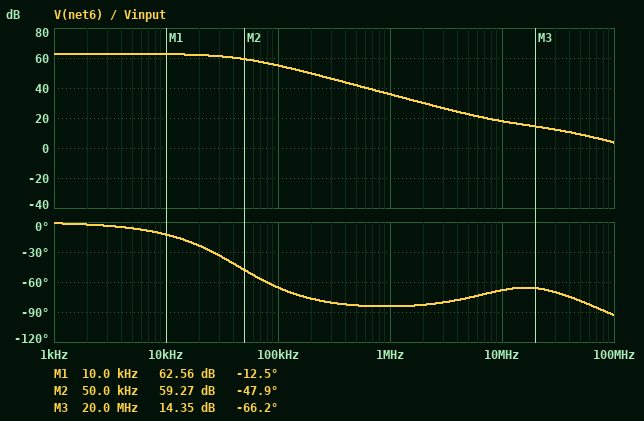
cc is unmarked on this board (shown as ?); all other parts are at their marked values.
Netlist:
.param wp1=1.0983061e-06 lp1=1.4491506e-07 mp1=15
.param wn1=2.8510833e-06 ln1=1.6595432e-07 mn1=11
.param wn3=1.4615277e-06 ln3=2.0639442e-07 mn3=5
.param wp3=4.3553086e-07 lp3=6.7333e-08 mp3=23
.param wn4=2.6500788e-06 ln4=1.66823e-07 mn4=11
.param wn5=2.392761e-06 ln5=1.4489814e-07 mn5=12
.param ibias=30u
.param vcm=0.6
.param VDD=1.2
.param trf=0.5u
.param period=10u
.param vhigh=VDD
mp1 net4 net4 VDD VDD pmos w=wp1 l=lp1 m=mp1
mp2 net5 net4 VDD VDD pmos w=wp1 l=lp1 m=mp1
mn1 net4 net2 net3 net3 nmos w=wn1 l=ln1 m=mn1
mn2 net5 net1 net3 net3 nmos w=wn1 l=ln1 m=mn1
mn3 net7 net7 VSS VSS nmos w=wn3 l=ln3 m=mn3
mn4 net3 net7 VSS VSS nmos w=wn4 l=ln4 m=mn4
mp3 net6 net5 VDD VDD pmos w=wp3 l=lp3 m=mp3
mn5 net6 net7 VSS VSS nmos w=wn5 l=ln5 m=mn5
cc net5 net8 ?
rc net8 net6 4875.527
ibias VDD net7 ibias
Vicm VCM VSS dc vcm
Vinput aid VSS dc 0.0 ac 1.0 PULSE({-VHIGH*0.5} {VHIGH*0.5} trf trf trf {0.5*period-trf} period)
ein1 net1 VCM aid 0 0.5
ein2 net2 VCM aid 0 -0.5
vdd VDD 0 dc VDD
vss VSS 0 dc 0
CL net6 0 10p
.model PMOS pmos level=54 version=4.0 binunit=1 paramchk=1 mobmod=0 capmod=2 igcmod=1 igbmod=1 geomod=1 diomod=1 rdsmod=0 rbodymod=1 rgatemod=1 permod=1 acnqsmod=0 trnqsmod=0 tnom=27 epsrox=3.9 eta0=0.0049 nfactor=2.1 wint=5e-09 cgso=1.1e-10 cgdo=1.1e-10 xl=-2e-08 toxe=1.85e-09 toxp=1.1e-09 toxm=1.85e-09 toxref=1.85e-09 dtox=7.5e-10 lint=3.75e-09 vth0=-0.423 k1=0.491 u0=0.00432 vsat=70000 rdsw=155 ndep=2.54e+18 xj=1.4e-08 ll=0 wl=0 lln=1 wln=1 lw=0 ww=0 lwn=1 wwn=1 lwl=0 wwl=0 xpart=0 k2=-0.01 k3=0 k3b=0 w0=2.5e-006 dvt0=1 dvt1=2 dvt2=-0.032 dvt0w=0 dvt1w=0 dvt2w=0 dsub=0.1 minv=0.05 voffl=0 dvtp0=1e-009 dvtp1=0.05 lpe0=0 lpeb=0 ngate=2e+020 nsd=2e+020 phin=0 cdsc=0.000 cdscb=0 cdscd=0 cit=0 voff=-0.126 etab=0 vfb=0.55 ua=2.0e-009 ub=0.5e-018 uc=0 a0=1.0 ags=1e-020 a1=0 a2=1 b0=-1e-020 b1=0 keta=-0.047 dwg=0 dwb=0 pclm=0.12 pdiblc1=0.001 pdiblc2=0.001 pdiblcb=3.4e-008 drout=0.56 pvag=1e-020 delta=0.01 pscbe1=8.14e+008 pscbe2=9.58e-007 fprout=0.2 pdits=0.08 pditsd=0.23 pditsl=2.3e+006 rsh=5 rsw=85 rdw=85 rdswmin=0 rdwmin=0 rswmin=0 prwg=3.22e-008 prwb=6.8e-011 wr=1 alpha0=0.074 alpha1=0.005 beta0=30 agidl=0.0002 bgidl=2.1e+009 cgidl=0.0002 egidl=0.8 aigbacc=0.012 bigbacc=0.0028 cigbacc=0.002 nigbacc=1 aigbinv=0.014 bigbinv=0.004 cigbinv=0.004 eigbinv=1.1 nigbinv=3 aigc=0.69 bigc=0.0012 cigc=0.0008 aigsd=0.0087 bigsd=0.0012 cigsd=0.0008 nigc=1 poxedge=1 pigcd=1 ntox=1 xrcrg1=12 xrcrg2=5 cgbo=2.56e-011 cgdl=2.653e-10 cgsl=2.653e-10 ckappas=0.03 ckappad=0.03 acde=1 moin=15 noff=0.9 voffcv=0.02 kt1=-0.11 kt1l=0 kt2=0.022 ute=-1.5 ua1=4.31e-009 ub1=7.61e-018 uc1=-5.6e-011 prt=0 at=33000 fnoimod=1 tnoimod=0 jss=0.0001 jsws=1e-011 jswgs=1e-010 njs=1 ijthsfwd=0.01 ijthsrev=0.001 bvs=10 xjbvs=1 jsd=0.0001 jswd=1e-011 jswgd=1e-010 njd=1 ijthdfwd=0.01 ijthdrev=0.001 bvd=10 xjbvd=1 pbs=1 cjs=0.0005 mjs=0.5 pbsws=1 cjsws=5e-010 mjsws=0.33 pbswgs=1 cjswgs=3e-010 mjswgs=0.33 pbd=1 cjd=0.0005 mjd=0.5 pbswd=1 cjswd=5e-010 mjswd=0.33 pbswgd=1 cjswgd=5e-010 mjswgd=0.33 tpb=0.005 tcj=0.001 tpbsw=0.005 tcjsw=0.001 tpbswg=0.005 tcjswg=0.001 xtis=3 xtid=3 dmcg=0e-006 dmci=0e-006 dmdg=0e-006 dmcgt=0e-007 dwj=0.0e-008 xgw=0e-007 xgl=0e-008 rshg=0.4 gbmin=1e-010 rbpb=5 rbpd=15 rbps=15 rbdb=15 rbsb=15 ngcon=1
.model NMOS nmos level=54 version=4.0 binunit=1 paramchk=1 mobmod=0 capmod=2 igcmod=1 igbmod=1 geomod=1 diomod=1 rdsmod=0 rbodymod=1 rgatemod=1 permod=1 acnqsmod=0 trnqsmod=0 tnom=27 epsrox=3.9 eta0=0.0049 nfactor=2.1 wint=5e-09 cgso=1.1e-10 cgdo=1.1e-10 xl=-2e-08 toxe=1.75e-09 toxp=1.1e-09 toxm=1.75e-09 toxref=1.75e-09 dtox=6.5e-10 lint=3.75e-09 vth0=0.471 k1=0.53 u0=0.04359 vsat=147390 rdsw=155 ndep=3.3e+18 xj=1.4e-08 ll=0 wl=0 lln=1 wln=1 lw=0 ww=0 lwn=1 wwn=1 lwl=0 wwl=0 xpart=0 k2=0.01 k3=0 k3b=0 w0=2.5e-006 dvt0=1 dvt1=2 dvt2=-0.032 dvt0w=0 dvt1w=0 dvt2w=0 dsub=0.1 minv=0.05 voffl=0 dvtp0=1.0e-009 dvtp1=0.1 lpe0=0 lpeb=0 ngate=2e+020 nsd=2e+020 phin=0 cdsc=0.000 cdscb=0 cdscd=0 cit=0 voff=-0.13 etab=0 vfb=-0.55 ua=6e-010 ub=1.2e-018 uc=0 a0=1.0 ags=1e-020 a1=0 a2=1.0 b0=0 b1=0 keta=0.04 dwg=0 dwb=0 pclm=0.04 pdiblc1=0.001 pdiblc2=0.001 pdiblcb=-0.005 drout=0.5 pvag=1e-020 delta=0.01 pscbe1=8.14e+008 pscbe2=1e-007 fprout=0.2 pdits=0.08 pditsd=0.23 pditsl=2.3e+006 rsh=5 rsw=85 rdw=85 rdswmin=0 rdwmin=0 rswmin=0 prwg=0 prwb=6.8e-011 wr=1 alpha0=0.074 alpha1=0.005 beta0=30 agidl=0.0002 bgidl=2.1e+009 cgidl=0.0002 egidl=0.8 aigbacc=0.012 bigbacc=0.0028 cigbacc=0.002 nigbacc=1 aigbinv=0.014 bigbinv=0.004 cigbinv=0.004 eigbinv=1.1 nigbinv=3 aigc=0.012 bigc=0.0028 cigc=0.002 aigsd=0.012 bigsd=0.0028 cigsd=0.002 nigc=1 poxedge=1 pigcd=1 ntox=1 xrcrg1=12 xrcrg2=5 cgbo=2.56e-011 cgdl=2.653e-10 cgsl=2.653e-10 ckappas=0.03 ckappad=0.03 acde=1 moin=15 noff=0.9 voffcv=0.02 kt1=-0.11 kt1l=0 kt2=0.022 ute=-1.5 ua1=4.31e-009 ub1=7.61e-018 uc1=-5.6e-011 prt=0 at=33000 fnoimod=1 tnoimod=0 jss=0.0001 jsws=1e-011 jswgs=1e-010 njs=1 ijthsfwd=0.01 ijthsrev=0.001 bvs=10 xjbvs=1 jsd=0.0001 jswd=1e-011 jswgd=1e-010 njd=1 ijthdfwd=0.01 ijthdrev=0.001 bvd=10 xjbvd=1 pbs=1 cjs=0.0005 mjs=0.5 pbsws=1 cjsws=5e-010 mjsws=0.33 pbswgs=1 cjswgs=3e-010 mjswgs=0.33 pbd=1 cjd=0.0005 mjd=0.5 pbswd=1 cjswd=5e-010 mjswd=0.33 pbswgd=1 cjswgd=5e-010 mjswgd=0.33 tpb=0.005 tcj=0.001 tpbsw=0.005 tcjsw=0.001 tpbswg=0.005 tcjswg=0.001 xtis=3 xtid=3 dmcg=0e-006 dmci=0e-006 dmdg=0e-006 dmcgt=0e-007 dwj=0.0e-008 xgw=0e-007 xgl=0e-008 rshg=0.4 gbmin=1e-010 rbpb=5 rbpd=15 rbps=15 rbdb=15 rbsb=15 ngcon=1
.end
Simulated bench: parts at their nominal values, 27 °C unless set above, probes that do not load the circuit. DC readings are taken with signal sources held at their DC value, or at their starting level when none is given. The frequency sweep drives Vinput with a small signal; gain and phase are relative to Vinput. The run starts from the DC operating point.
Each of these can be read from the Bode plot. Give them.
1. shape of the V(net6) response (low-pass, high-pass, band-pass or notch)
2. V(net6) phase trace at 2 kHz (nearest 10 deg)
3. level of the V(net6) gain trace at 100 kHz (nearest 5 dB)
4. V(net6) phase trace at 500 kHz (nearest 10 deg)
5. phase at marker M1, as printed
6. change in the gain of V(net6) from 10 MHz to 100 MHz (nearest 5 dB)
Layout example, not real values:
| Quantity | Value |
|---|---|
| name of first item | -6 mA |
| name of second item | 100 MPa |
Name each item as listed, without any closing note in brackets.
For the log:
| Quantity | Value |
|---|---|
| shape of the V(net6) response | low-pass |
| V(net6) phase trace at 2 kHz | 0 deg |
| level of the V(net6) gain trace at 100 kHz | 55 dB |
| V(net6) phase trace at 500 kHz | -80 deg |
| phase at marker M1, as printed | -12.5 deg |
| change in the gain of V(net6) from 10 MHz to 100 MHz | -15 dB |
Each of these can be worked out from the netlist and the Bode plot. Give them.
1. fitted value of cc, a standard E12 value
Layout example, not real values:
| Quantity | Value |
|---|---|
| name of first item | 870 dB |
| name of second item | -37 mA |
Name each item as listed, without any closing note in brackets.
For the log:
| Quantity | Value |
|---|---|
| fitted value of cc, a standard E12 value | 3.3 pF |
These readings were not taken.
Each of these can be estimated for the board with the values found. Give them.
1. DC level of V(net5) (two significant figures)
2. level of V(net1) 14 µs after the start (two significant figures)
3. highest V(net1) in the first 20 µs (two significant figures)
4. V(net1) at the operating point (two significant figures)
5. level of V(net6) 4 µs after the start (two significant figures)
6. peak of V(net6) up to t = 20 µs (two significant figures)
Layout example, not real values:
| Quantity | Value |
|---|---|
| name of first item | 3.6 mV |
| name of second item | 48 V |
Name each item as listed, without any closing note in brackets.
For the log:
| Quantity | Value |
|---|---|
| DC level of V(net5) | 640 mV |
| level of V(net1) 14 µs after the start | 900 mV |
| highest V(net1) in the first 20 µs | 900 mV |
| V(net1) at the operating point | 600 mV |
| level of V(net6) 4 µs after the start | 1.2 V |
| peak of V(net6) up to t = 20 µs | 1.2 V |
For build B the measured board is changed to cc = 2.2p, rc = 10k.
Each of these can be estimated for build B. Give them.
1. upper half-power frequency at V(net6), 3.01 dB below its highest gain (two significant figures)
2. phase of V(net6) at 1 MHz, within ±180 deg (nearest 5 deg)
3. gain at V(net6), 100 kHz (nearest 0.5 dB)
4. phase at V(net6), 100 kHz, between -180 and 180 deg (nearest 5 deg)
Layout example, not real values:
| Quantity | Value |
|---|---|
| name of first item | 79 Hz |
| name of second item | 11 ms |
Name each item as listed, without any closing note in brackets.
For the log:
| Quantity | Value |
|---|---|
| upper half-power frequency at V(net6), 3.01 dB below its highest gain | 66 kHz |
| phase of V(net6) at 1 MHz, within ±180 deg | -80 deg |
| gain at V(net6), 100 kHz | 57.5 dB |
| phase at V(net6), 100 kHz, between -180 and 180 deg | -55 deg |
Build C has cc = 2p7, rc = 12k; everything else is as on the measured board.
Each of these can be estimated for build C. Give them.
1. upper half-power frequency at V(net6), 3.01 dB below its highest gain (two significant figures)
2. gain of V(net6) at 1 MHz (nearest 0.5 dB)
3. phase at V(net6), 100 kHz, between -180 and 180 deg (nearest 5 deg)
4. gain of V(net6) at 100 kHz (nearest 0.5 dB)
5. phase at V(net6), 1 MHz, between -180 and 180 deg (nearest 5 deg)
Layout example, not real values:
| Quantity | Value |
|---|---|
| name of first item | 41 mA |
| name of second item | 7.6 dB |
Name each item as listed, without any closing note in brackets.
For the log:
| Quantity | Value |
|---|---|
| upper half-power frequency at V(net6), 3.01 dB below its highest gain | 54 kHz |
| gain of V(net6) at 1 MHz | 37.5 dB |
| phase at V(net6), 100 kHz, between -180 and 180 deg | -60 deg |
| gain of V(net6) at 100 kHz | 56.5 dB |
| phase at V(net6), 1 MHz, between -180 and 180 deg | -80 deg |
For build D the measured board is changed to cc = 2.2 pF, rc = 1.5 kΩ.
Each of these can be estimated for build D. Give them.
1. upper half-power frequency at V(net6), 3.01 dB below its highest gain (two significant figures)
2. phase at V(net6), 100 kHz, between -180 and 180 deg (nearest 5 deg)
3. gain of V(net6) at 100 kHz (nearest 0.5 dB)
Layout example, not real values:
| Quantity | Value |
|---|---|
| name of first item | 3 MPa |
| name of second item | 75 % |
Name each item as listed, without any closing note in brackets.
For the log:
| Quantity | Value |
|---|---|
| upper half-power frequency at V(net6), 3.01 dB below its highest gain | 67 kHz |
| phase at V(net6), 100 kHz, between -180 and 180 deg | -55 deg |
| gain of V(net6) at 100 kHz | 57.5 dB |
